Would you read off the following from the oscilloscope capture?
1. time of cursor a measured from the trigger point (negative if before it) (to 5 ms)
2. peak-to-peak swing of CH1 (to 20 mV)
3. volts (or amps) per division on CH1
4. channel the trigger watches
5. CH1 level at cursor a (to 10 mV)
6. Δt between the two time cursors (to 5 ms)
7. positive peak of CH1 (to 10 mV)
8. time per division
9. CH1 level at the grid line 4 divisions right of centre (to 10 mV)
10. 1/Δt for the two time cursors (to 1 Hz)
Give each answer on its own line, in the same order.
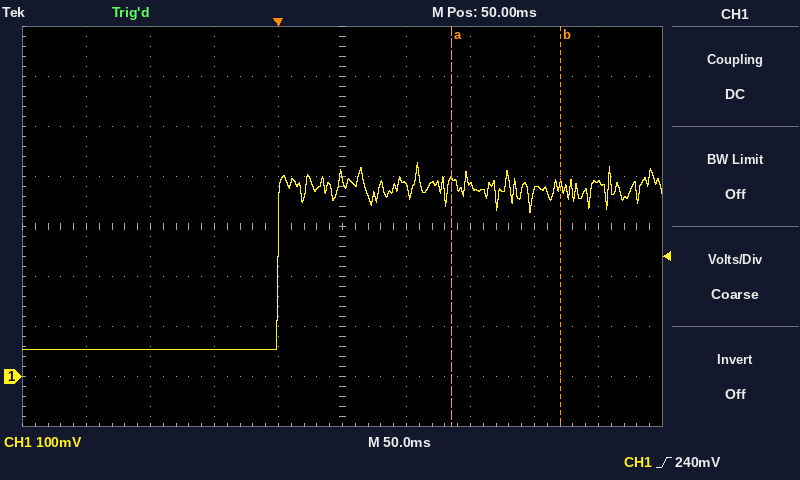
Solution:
+135 ms
380 mV
100 mV
CH1
390 mV
85 ms
430 mV
50 ms
390 mV
12 Hz
